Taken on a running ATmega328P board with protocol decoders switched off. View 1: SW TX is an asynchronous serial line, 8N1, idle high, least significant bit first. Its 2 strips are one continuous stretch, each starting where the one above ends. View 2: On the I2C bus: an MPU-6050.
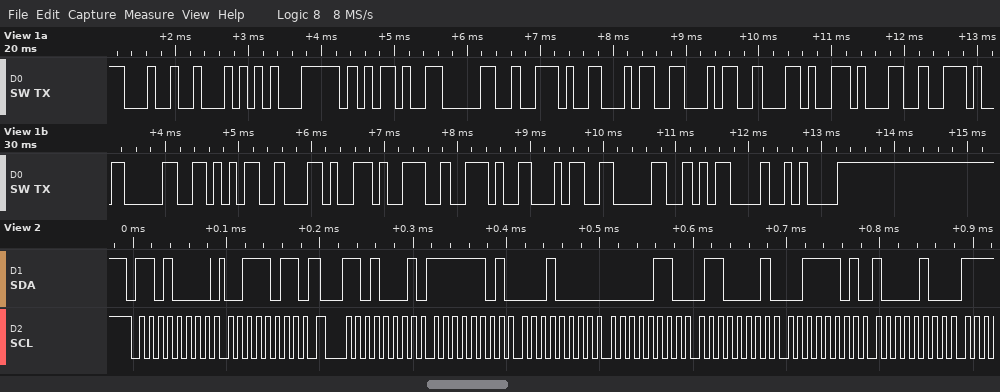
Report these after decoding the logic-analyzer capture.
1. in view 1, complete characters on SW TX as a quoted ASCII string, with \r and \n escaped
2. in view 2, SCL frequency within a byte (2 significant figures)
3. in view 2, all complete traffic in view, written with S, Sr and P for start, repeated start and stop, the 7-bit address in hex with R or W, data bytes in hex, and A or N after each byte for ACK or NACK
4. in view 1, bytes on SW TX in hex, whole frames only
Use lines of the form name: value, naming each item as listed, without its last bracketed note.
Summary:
in view 1, complete characters on SW TX as a quoted ASCII string, with \r and \n escaped: "$T|-0.44,1.05,9.40\r\n"
in view 2, SCL frequency within a byte: 100 kHz
in view 2, all complete traffic in view, written with S, Sr and P for start, repeated start and stop, the 7-bit address in hex with R or W, data bytes in hex, and A or N after each byte for ACK or NACK: S 68W A 3B A Sr 68R A FD A 10 A 06 A 61 A 3D A 84 A
in view 1, bytes on SW TX in hex, whole frames only: 24 54 7C 2D 30 2E 34 34 2C 31 2E 30 35 2C 39 2E 34 30 0D 0A
